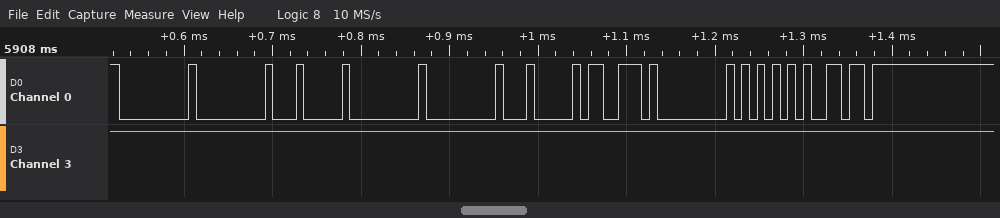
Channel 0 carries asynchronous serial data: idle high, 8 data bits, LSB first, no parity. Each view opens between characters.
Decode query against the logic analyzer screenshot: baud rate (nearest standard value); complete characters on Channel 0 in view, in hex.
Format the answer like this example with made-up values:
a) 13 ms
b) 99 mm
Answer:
a) 115200 baud
b) 00, 00, 04, 00, 00, 04, 73, 00, 55, B6
